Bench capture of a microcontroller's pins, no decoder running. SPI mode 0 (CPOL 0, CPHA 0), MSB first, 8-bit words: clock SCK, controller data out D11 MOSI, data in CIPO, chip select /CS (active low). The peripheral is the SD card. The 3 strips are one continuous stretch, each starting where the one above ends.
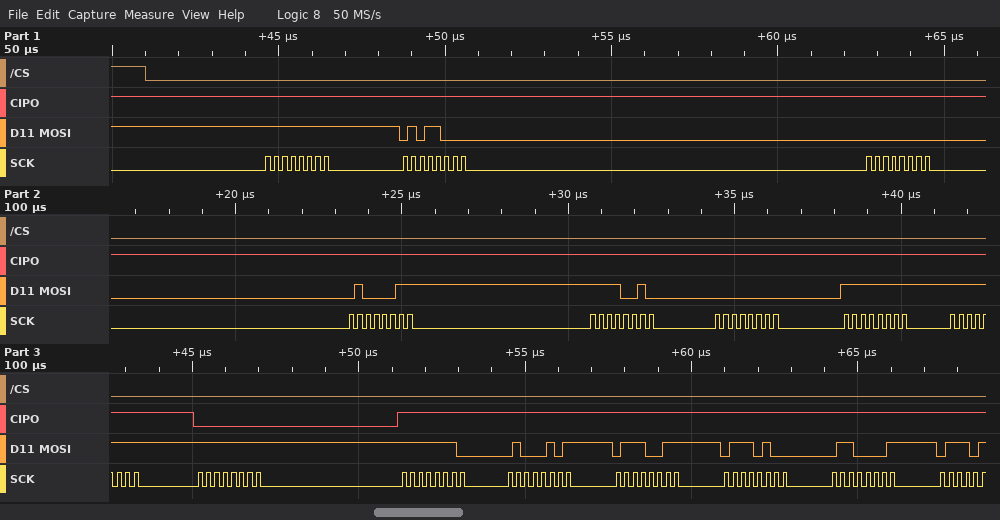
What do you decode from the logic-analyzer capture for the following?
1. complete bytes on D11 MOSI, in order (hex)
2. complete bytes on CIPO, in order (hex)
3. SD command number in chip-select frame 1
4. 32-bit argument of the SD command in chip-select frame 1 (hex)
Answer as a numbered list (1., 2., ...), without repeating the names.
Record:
1. FF 58 00 43 F2 00 FF FF FF FE 45 73 74 61
2. FF FF FF FF FF FF FF FF 00 FF FF FF FF FF
3. CMD24
4. 0x0043F200
